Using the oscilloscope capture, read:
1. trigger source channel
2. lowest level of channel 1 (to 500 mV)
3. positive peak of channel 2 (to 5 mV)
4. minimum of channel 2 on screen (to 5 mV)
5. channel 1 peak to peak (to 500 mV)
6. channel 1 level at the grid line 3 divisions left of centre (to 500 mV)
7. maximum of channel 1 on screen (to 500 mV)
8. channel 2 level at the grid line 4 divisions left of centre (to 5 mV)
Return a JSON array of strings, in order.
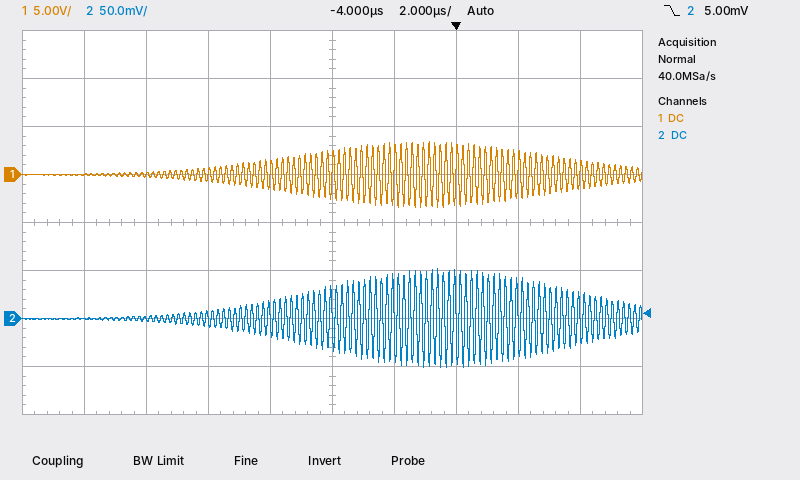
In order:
["channel 2", "-3.5 V", "50 mV", "-50 mV", "7.0 V", "0.0 V", "3.5 V", "0 mV"]
